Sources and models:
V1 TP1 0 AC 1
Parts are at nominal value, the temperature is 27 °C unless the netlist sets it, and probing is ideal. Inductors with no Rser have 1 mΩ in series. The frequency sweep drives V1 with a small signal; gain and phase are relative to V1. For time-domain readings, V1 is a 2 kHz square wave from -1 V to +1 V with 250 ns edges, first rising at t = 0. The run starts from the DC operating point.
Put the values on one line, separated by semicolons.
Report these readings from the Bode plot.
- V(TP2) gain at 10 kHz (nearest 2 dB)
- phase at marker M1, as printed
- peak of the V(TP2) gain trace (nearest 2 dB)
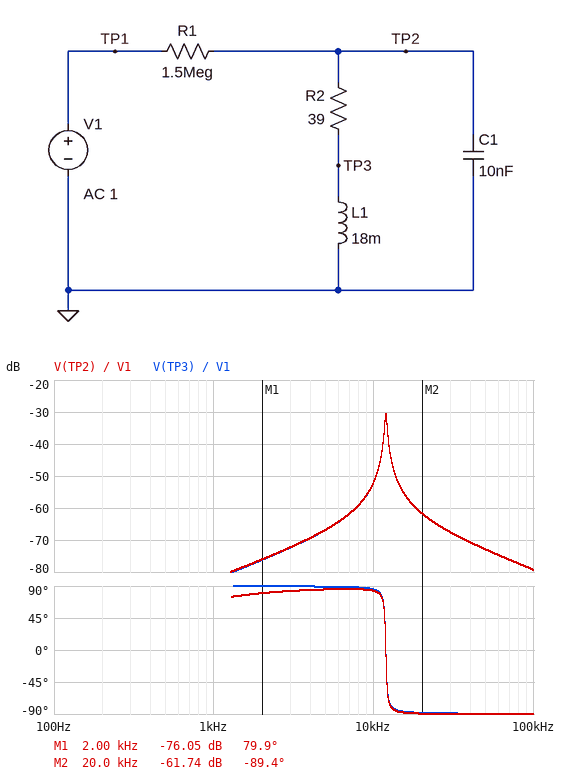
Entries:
-52 dB; 79.9 deg; -30 dB
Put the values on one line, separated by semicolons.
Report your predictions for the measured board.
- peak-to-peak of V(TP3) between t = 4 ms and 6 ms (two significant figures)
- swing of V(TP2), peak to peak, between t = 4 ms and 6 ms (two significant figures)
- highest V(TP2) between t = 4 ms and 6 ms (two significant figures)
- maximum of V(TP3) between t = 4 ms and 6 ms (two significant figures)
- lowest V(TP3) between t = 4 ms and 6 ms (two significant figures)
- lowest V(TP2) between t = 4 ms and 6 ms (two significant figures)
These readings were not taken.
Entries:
2.0 mV; 2.1 mV; 1.0 mV; 1.0 mV; -1.0 mV; -1.0 mV
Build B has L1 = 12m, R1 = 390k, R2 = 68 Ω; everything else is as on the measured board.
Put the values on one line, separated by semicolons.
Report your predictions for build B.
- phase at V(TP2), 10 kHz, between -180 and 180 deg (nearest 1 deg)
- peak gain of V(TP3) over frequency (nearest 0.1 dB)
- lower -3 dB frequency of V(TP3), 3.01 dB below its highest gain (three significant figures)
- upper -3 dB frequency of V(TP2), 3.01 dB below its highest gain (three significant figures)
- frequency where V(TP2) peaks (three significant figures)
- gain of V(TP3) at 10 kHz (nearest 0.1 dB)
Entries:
80 deg; -27.3 dB; 14.1 kHz; 15.0 kHz; 14.5 kHz; -48.7 dB
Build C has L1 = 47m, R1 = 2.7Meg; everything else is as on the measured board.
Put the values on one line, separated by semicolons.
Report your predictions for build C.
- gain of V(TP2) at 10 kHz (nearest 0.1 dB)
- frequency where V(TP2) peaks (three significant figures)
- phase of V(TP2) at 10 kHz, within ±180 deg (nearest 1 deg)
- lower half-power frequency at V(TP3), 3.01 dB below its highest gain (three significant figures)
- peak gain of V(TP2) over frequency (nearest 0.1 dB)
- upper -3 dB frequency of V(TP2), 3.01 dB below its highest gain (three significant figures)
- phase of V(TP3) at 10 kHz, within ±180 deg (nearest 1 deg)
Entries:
-57.9 dB; 7.34 kHz; -89 deg; 7.27 kHz; -27.4 dB; 7.41 kHz; -88 deg
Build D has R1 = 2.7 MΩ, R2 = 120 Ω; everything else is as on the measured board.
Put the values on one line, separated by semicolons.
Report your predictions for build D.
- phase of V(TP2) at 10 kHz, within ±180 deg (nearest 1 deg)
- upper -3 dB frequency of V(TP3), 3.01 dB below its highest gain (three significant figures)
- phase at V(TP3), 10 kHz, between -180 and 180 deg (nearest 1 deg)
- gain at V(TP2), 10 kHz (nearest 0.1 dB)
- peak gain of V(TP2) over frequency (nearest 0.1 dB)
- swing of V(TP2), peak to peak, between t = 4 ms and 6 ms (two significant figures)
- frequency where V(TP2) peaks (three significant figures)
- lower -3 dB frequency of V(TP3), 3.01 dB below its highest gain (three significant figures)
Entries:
69 deg; 12.4 kHz; 75 deg; -57.0 dB; -45.1 dB; 1.4 mV; 11.9 kHz; 11.3 kHz
